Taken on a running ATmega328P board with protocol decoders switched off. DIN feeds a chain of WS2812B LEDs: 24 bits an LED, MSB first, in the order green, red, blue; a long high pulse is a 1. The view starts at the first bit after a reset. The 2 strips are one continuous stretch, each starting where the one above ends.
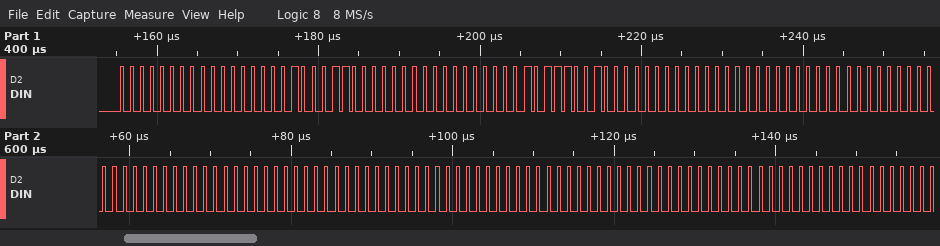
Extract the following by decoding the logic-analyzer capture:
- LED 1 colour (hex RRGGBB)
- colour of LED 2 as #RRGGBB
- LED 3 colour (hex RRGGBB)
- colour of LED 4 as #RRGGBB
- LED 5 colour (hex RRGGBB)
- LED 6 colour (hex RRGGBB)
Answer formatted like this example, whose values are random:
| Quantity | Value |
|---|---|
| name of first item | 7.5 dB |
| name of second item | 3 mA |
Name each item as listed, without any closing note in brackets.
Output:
| Quantity | Value |
|---|---|
| LED 1 colour | #000046 |
| colour of LED 2 as #RRGGBB | #0000B9 |
| LED 3 colour | #000000 |
| colour of LED 4 as #RRGGBB | #000000 |
| LED 5 colour | #000000 |
| LED 6 colour | #000000 |
